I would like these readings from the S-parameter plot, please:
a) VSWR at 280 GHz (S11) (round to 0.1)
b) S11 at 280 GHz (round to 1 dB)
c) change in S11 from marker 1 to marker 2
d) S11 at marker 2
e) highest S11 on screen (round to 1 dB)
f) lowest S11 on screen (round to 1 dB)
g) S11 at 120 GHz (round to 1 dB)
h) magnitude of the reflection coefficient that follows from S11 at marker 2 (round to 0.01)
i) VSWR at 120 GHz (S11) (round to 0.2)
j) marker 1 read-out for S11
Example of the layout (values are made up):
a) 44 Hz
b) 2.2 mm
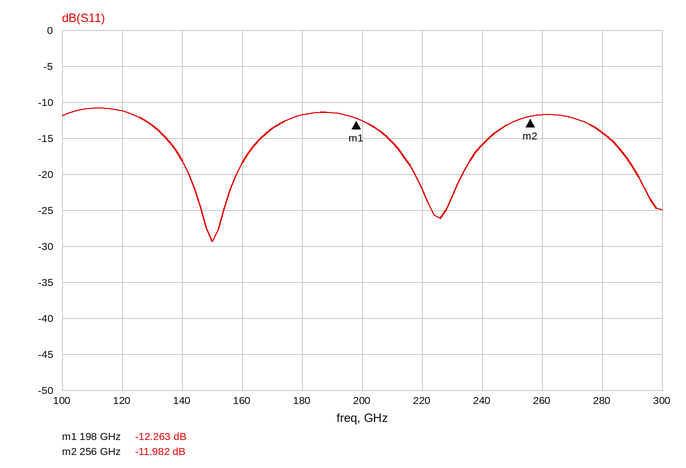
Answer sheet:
a) 1.5
b) -14 dB
c) 0.281 dB
d) -11.982 dB
e) -11 dB
f) -29 dB
g) -11 dB
h) 0.25
i) 1.8
j) -12.263 dB
